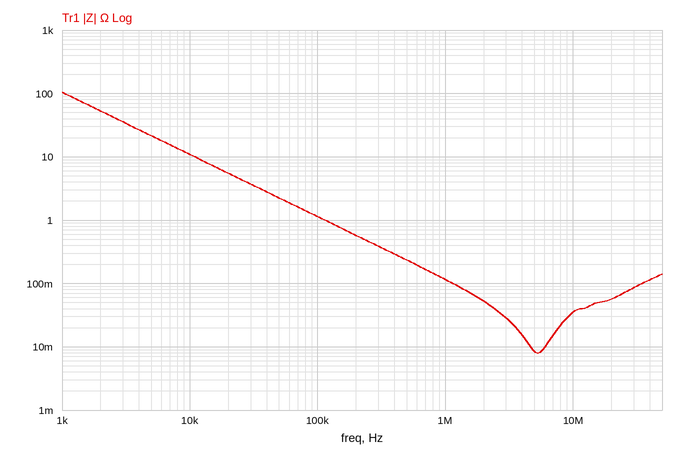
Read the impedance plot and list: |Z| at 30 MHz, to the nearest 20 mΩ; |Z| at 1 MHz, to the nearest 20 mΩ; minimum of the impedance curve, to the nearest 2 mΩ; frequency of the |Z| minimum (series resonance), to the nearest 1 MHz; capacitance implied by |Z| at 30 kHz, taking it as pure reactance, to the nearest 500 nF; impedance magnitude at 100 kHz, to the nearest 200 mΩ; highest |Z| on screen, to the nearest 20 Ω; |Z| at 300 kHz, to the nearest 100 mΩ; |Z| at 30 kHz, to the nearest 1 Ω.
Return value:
80 mΩ
120 mΩ
8 mΩ
5 MHz
1.5 µF
1.2 Ω
100 Ω
400 mΩ
4 Ω
